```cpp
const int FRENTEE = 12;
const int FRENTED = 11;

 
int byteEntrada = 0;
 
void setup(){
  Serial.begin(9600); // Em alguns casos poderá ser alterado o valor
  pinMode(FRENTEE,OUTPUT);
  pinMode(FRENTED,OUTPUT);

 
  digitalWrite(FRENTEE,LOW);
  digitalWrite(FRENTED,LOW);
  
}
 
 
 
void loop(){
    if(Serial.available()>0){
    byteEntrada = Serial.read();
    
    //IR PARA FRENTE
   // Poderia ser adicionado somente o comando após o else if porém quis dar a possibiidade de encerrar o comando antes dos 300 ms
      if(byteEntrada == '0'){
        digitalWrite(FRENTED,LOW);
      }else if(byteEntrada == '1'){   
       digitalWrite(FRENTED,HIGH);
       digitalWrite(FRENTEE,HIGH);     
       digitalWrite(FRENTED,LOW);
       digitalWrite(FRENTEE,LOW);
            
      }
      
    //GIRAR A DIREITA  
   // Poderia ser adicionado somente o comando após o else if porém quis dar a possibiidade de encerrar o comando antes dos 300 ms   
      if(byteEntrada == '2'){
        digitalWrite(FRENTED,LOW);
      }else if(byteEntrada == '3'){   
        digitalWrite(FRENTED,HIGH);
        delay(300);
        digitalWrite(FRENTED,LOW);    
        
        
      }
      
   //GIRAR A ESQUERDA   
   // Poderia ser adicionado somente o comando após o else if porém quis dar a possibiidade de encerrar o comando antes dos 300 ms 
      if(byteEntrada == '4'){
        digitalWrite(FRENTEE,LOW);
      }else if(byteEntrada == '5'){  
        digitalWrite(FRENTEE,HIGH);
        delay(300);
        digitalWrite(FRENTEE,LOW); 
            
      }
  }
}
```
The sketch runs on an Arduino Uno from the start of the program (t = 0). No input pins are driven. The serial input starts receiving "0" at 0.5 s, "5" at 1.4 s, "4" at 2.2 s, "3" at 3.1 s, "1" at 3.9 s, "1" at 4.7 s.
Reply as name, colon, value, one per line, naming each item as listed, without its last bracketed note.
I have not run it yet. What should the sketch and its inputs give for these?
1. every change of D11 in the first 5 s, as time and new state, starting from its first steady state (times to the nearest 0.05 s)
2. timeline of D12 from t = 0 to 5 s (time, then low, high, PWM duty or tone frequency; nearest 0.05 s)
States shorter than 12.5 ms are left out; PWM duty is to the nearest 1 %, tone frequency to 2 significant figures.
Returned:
every change of D11 in the first 5 s, as time and new state, starting from its first steady state: 0 s low; 3.1 s high; 3.4 s low
timeline of D12 from t = 0 to 5 s: 0 s low; 1.4 s high; 1.7 s low
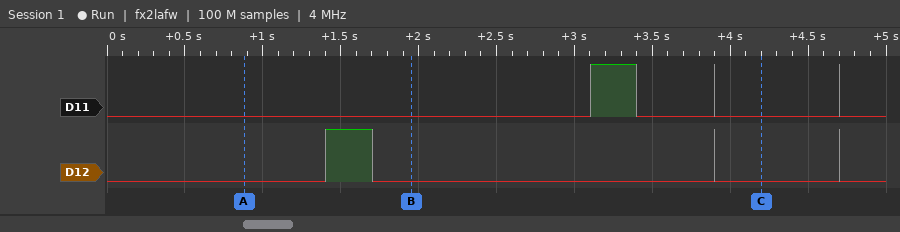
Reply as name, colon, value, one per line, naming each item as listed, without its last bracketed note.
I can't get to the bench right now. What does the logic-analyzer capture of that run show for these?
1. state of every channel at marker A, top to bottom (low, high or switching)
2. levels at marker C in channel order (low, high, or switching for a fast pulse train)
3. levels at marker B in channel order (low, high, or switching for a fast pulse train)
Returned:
state of every channel at marker A, top to bottom: D11 low, D12 low
levels at marker C in channel order: D11 low, D12 low
levels at marker B in channel order: D11 low, D12 low
